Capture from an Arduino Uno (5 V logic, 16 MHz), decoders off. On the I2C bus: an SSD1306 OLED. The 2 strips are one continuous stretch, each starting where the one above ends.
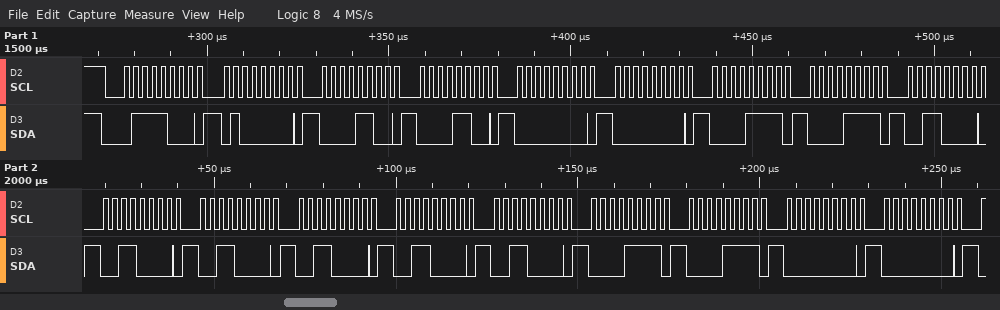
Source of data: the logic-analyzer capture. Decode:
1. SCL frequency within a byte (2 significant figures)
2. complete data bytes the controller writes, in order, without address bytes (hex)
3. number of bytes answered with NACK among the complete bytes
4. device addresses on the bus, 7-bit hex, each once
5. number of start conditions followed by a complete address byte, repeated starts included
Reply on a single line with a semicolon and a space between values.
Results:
400 kHz; 40 0C 0C 00 00 0F 0F 30 30 30 30 30 30 0F 0F 00 00; 0; 0x3C; 1
